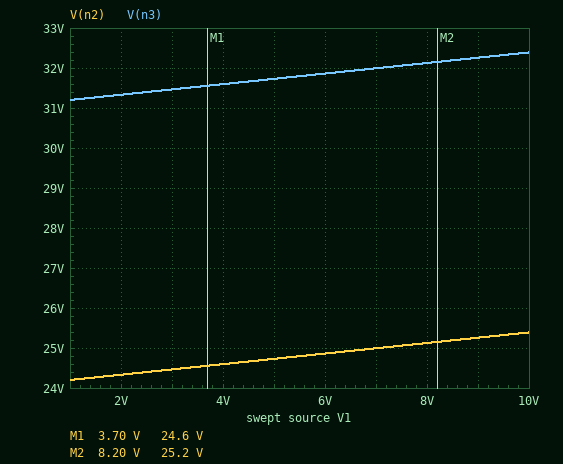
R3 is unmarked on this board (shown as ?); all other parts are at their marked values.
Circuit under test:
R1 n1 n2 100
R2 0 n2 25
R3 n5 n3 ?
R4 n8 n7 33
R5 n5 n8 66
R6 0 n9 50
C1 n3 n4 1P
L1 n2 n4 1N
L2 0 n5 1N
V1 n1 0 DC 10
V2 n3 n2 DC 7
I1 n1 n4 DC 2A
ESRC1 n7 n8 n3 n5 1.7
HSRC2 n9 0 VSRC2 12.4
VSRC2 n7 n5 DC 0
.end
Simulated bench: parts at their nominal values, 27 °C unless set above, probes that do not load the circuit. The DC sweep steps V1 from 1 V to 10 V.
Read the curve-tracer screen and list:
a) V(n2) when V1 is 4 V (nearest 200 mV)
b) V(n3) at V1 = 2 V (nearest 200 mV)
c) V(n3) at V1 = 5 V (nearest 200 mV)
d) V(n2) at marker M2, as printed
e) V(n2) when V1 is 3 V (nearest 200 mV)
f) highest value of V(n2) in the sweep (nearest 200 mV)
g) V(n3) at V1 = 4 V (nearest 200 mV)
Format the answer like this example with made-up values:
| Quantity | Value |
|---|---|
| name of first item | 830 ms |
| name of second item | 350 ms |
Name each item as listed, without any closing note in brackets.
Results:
| Quantity | Value |
|---|---|
| V(n2) when V1 is 4 V | 24.6 V |
| V(n3) at V1 = 2 V | 31.4 V |
| V(n3) at V1 = 5 V | 31.8 V |
| V(n2) at marker M2, as printed | 25.2 V |
| V(n2) when V1 is 3 V | 24.4 V |
| highest value of V(n2) in the sweep | 25.4 V |
| V(n3) at V1 = 4 V | 31.6 V |
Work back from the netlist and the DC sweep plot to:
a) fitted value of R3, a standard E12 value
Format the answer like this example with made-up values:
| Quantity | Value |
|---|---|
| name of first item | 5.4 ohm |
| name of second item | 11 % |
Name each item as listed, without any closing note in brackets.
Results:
| Quantity | Value |
|---|---|
| fitted value of R3, a standard E12 value | 39 Ω |
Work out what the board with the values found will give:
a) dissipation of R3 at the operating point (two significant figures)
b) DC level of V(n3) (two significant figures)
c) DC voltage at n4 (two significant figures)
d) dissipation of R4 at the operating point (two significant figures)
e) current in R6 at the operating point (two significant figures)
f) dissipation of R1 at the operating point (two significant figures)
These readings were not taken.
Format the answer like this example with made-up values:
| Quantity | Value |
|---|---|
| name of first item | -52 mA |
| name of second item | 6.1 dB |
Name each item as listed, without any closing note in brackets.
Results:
| Quantity | Value |
|---|---|
| dissipation of R3 at the operating point | 27 W |
| DC level of V(n3) | 32 V |
| DC voltage at n4 | 25 V |
| dissipation of R4 at the operating point | 92 W |
| current in R6 at the operating point | 210 mA |
| dissipation of R1 at the operating point | 2.4 W |
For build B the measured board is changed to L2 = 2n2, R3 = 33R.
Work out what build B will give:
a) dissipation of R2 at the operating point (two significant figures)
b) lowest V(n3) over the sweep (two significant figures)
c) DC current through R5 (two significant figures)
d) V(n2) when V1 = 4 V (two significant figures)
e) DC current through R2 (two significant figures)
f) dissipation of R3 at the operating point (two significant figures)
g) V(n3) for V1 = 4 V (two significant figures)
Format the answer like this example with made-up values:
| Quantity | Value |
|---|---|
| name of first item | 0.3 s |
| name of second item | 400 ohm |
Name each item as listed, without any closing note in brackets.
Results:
| Quantity | Value |
|---|---|
| dissipation of R2 at the operating point | 22 W |
| lowest V(n3) over the sweep | 29 V |
| DC current through R5 | 790 mA |
| V(n2) when V1 = 4 V | 23 V |
| DC current through R2 | 940 mA |
| dissipation of R3 at the operating point | 28 W |
| V(n3) for V1 = 4 V | 30 V |
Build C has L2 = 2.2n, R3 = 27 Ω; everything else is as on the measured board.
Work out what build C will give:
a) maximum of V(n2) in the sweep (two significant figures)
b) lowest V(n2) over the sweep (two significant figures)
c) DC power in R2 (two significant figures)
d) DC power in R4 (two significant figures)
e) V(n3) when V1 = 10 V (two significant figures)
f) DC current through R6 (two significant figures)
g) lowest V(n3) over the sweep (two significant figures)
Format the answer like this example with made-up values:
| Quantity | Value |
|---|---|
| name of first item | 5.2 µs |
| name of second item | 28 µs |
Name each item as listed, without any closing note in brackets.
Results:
| Quantity | Value |
|---|---|
| maximum of V(n2) in the sweep | 21 V |
| lowest V(n2) over the sweep | 20 V |
| DC power in R2 | 18 W |
| DC power in R4 | 69 W |
| V(n3) when V1 = 10 V | 28 V |
| DC current through R6 | 180 mA |
| lowest V(n3) over the sweep | 27 V |
